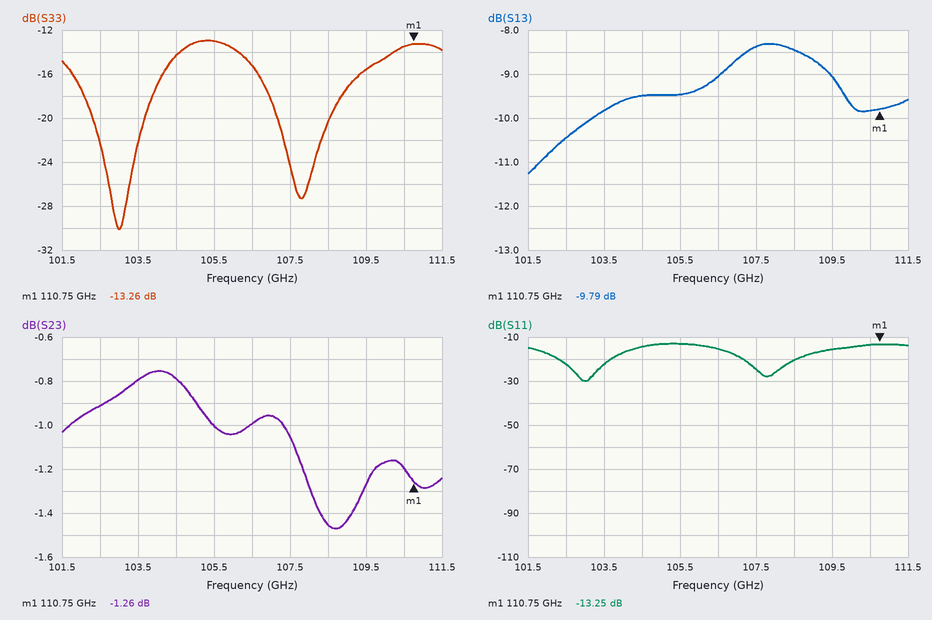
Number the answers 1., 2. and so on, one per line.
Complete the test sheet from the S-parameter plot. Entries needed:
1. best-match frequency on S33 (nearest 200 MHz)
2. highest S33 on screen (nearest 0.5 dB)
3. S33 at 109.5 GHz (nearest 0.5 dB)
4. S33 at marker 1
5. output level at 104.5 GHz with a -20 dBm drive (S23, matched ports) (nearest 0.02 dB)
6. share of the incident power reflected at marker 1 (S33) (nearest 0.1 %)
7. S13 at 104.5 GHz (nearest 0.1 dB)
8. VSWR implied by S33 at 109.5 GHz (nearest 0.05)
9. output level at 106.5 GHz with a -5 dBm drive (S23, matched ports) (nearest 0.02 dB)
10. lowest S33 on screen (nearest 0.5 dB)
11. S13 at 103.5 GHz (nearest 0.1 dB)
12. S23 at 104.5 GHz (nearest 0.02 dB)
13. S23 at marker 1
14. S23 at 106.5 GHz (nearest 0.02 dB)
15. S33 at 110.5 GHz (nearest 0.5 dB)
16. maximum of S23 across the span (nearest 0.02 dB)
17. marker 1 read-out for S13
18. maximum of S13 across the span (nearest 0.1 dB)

1. 103.0 GHz
2. -13.0 dB
3. -15.5 dB
4. -13.26 dB
5. -20.78 dBm
6. 4.7 %
7. -9.5 dB
8. 1.40
9. -6.00 dBm
10. -30.0 dB
11. -9.8 dB
12. -0.78 dB
13. -1.26 dB
14. -1.00 dB
15. -13.5 dB
16. -0.76 dB
17. -9.79 dB
18. -8.3 dB
